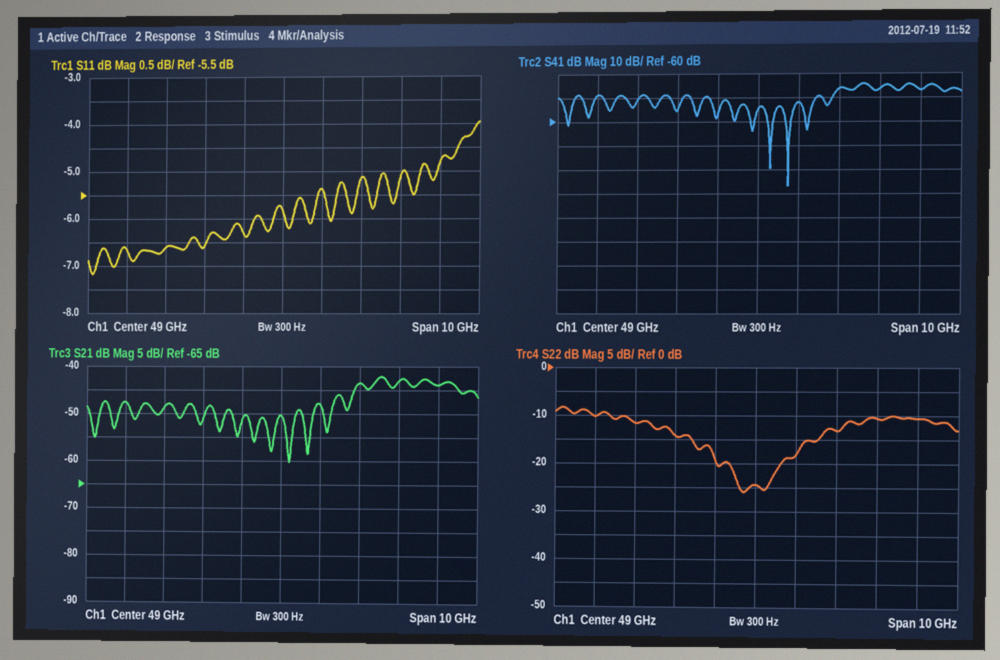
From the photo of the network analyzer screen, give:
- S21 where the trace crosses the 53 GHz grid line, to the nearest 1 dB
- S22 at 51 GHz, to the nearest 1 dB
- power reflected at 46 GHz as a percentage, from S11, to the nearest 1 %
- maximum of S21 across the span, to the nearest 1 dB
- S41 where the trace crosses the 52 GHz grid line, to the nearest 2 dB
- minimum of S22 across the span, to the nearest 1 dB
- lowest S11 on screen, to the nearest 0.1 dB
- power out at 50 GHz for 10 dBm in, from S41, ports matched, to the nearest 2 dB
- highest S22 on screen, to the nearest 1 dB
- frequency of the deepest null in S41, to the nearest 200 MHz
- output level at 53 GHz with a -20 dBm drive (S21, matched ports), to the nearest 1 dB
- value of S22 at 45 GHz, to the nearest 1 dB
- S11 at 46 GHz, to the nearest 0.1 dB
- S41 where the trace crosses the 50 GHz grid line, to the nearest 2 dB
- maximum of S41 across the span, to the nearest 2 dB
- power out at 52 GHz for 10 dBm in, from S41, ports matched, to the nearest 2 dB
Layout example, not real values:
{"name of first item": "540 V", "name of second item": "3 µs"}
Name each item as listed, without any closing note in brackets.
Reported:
{"S21 where the trace crosses the 53 GHz grid line, to the nearest 1 dB": "-44 dB", "S22 at 51 GHz, to the nearest 1 dB": "-13 dB", "power reflected at 46 GHz as a percentage, from S11, to the nearest 1 %": "22 %", "maximum of S21 across the span, to the nearest 1 dB": "-42 dB", "S41 where the trace crosses the 52 GHz grid line, to the nearest 2 dB": "-46 dB", "minimum of S22 across the span, to the nearest 1 dB": "-26 dB", "lowest S11 on screen, to the nearest 0.1 dB": "-7.2 dB", "power out at 50 GHz for 10 dBm in, from S41, ports matched, to the nearest 2 dB": "-42 dBm", "highest S22 on screen, to the nearest 1 dB": "-8 dB", "frequency of the deepest null in S41, to the nearest 200 MHz": "49.8 GHz", "output level at 53 GHz with a -20 dBm drive (S21, matched ports), to the nearest 1 dB": "-64 dBm", "value of S22 at 45 GHz, to the nearest 1 dB": "-10 dB", "S11 at 46 GHz, to the nearest 0.1 dB": "-6.6 dB", "S41 where the trace crosses the 50 GHz grid line, to the nearest 2 dB": "-52 dB", "maximum of S41 across the span, to the nearest 2 dB": "-44 dB", "power out at 52 GHz for 10 dBm in, from S41, ports matched, to the nearest 2 dB": "-36 dBm"}
